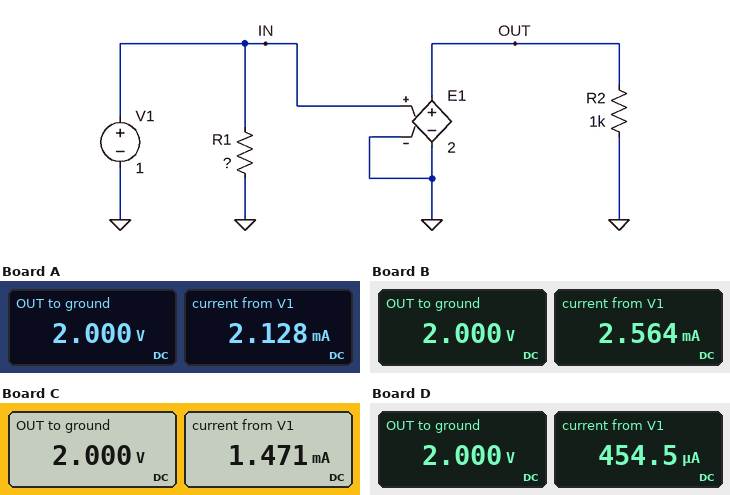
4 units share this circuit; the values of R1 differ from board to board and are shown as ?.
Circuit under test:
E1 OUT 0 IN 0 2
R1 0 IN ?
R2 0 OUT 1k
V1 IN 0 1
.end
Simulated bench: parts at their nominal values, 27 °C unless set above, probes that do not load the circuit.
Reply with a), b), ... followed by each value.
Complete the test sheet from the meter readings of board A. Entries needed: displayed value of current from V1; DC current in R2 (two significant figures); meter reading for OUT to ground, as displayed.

a) 2.128 mA
b) 2.0 mA
c) 2.000 V
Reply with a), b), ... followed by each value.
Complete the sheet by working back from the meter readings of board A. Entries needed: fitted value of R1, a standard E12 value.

a) 470 Ω
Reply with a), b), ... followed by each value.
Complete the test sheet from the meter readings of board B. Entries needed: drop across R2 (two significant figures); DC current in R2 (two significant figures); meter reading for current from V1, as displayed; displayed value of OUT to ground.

a) 2.0 V
b) 2.0 mA
c) 2.564 mA
d) 2.000 V
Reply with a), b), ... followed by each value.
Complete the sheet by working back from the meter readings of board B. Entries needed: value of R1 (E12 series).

a) 390 Ω
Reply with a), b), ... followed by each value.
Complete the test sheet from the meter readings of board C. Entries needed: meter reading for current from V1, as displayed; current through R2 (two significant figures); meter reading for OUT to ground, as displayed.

a) 1.471 mA
b) 2.0 mA
c) 2.000 V
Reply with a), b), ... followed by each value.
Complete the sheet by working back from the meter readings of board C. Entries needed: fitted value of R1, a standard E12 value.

a) 680 Ω
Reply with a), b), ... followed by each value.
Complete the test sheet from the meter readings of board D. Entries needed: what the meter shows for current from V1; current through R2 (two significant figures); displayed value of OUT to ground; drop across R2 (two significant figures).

a) 454.5 µA
b) 2.0 mA
c) 2.000 V
d) 2.0 V
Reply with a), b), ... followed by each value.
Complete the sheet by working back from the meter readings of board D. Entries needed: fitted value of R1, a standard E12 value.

a) 2.2 kΩ
